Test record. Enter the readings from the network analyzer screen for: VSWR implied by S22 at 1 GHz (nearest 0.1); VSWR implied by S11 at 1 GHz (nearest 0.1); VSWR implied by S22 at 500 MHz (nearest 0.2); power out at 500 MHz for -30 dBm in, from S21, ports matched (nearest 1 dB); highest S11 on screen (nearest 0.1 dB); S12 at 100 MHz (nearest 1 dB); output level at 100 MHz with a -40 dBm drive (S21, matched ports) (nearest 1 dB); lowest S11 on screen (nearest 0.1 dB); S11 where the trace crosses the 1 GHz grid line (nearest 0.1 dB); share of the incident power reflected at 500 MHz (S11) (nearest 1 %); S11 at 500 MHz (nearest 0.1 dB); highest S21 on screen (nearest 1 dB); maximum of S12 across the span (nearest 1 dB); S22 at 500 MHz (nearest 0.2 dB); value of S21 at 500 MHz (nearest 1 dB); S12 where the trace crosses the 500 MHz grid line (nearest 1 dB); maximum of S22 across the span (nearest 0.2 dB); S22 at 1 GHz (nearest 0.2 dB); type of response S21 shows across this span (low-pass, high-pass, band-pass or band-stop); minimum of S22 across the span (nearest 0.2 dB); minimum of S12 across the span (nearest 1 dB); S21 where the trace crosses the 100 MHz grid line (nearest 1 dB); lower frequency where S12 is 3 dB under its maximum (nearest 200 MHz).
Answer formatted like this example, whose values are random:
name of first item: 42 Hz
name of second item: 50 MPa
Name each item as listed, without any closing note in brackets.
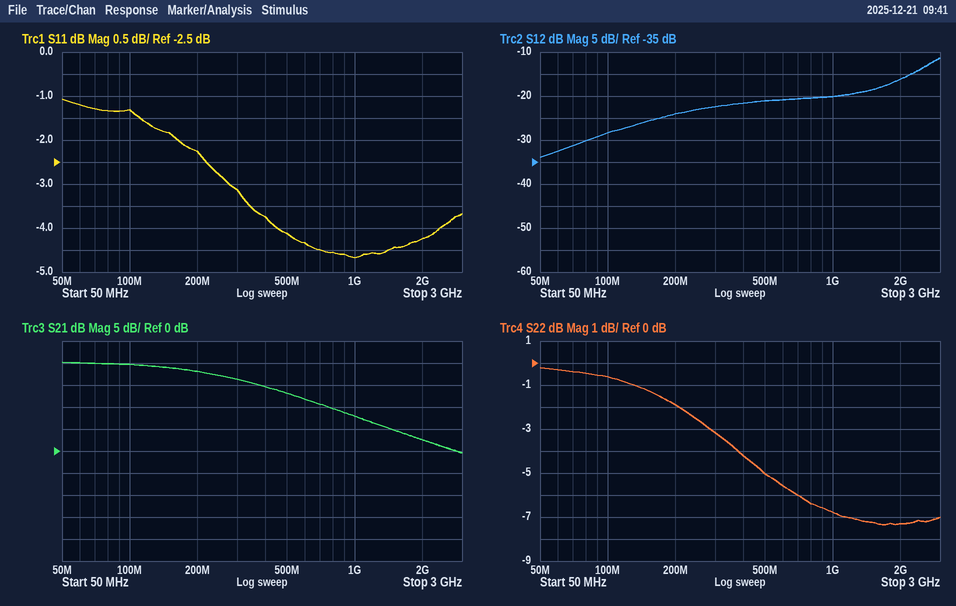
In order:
VSWR implied by S22 at 1 GHz: 2.7
VSWR implied by S11 at 1 GHz: 3.8
VSWR implied by S22 at 500 MHz: 3.6
power out at 500 MHz for -30 dBm in, from S21, ports matched: -17 dBm
highest S11 on screen: -1.1 dB
S12 at 100 MHz: -28 dB
output level at 100 MHz with a -40 dBm drive (S21, matched ports): -20 dBm
lowest S11 on screen: -4.7 dB
S11 where the trace crosses the 1 GHz grid line: -4.7 dB
share of the incident power reflected at 500 MHz (S11): 39 %
S11 at 500 MHz: -4.1 dB
highest S21 on screen: 20 dB
maximum of S12 across the span: -11 dB
S22 at 500 MHz: -5.0 dB
value of S21 at 500 MHz: 13 dB
S12 where the trace crosses the 500 MHz grid line: -21 dB
maximum of S22 across the span: -0.2 dB
S22 at 1 GHz: -6.8 dB
type of response S21 shows across this span: low-pass
minimum of S22 across the span: -7.4 dB
minimum of S12 across the span: -34 dB
S21 where the trace crosses the 100 MHz grid line: 20 dB
lower frequency where S12 is 3 dB under its maximum: 2.4 GHz
